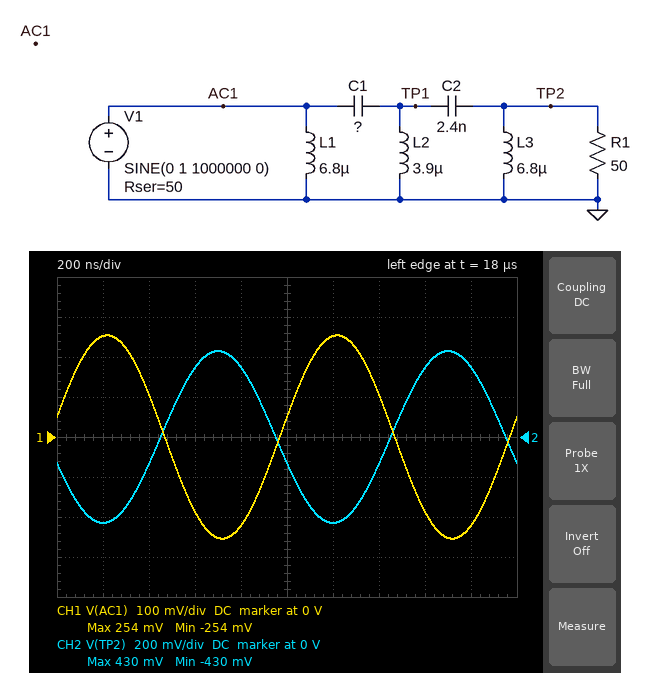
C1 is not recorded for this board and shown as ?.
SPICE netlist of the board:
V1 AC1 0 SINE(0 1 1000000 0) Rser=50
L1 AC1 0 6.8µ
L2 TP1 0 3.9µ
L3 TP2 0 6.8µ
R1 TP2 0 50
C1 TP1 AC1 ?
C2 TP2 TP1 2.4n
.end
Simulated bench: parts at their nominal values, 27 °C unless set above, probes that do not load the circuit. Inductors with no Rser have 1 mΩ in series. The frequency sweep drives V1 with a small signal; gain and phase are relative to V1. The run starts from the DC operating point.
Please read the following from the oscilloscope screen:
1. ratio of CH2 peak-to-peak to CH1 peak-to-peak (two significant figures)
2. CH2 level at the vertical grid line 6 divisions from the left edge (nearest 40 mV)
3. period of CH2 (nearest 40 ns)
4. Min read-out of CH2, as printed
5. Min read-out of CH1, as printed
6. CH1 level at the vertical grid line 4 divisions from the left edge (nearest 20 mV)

1.7
-440 mV
1.00 µs
-430 mV
-254 mV
-220 mV
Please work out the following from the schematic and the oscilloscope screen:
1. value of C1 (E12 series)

3.9 nF
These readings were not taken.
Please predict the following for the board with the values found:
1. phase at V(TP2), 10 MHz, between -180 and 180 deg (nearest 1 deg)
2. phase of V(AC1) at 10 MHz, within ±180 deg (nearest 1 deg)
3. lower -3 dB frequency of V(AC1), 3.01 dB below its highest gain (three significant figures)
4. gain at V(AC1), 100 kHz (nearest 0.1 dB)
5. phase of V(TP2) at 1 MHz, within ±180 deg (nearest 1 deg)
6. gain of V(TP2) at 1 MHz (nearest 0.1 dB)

19 deg
6 deg
572 kHz
-21.3 dB
-162 deg
-7.3 dB
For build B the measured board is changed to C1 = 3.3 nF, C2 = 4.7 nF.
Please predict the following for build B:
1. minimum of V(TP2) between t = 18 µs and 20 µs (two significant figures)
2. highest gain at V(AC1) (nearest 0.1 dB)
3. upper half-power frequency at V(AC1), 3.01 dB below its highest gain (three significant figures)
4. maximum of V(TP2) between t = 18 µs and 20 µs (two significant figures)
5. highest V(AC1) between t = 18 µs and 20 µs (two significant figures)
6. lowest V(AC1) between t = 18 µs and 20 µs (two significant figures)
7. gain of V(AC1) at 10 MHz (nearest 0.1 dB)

-480 mV
-3.0 dB
1.27 MHz
480 mV
650 mV
-650 mV
-6.3 dB
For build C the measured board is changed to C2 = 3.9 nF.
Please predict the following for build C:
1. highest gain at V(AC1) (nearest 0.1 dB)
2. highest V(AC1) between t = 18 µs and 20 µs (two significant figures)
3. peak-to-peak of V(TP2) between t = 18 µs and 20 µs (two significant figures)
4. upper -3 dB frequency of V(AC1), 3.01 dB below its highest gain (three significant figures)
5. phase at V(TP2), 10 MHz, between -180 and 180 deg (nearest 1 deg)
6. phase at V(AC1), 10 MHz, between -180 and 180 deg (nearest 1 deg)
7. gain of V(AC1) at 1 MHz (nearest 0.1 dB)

-1.8 dB
510 mV
1.0 V
742 kHz
17 deg
8 deg
-5.9 dB
